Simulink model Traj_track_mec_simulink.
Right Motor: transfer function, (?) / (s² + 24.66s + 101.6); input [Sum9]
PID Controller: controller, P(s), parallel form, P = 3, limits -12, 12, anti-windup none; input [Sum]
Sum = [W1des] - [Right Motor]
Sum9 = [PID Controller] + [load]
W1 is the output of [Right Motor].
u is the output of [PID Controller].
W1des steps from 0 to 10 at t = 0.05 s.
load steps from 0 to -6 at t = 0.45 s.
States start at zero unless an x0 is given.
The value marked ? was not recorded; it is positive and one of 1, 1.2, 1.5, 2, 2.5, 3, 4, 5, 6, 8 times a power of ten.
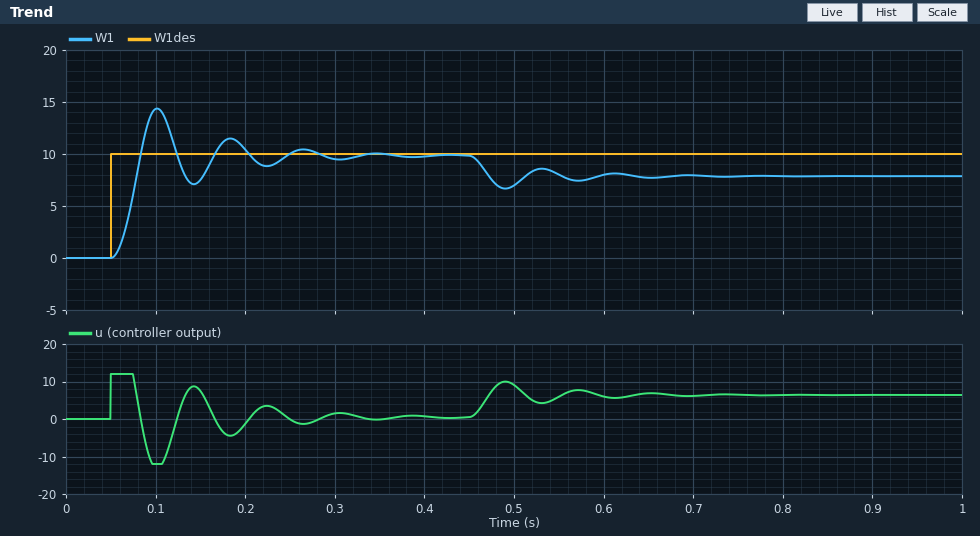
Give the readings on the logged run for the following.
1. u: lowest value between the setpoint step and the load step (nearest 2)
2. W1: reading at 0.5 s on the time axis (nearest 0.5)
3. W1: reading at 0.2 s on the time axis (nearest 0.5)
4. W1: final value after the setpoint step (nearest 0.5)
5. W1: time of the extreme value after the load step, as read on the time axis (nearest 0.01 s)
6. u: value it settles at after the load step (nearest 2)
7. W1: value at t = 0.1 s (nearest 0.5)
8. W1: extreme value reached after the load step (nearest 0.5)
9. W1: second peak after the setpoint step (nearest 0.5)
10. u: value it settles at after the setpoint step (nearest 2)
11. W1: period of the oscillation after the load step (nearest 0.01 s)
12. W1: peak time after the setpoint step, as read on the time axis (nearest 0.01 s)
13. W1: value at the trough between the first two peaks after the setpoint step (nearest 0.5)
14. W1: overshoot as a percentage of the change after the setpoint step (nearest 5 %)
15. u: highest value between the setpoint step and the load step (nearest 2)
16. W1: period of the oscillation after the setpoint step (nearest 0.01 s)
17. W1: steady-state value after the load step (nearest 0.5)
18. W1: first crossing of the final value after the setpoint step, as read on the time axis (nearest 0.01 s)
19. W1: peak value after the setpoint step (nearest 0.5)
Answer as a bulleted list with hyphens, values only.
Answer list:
- -12
- 7.0
- 10.5
- 10.0
- 0.49 s
- 6
- 14.5
- 6.5
- 11.5
- 0
- 0.08 s
- 0.10 s
- 7.0
- 45 %
- 12
- 0.08 s
- 8.0
- 0.08 s
- 14.5
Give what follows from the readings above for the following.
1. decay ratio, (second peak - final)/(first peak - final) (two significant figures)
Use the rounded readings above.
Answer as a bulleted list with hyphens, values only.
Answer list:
- 0.33
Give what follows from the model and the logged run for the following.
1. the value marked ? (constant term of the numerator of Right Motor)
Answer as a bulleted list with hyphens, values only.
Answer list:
- 2000
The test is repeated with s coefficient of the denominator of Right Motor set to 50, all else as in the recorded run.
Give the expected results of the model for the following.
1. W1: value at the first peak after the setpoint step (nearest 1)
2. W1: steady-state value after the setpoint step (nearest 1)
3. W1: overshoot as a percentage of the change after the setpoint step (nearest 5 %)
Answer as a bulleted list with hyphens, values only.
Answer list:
- 12
- 10
- 25 %
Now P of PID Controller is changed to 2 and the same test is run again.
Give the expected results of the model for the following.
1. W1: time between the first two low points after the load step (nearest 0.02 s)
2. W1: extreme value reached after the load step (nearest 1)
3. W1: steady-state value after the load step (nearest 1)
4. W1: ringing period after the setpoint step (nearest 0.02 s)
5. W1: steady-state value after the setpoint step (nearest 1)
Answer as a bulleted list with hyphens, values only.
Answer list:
- 0.10 s
- 5
- 7
- 0.10 s
- 10
